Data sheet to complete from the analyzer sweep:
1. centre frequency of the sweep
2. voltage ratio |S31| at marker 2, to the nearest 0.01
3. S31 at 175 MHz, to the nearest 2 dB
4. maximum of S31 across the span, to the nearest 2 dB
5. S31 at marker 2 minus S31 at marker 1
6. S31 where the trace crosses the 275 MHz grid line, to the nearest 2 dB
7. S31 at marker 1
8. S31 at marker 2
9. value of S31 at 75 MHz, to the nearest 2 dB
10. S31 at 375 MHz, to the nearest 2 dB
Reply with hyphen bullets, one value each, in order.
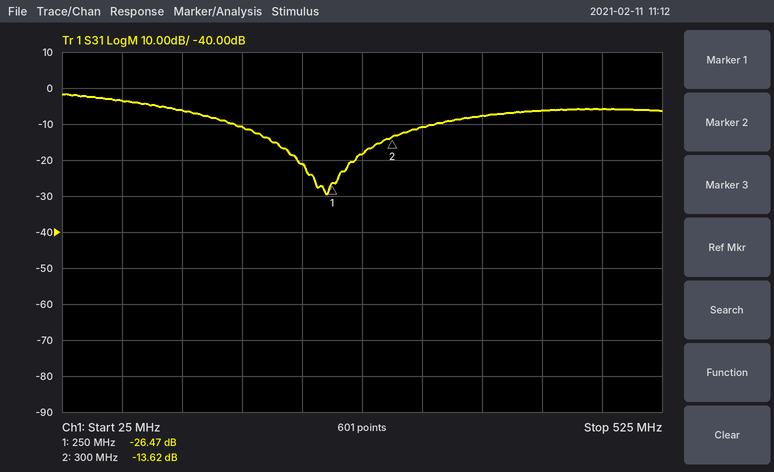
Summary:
- 275 MHz
- 0.21
- -10 dB
- -2 dB
- 12.85 dB
- -18 dB
- -26.47 dB
- -13.62 dB
- -4 dB
- -8 dB
